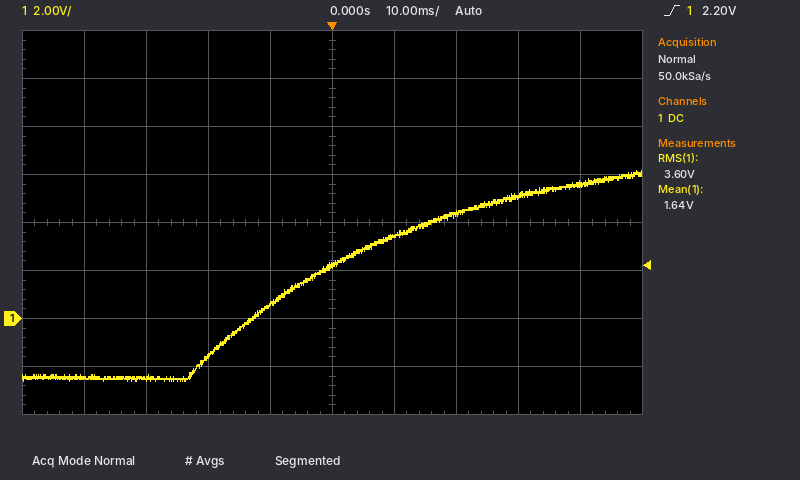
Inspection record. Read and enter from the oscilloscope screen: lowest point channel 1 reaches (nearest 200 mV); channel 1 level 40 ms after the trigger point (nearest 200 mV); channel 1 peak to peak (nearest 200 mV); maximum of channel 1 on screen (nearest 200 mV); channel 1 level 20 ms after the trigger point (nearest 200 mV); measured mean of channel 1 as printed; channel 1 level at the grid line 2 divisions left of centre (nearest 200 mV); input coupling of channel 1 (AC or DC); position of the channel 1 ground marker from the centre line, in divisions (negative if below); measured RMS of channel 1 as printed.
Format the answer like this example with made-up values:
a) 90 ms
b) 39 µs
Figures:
a) -2.6 V
b) 5.6 V
c) 8.8 V
d) 6.2 V
e) 4.4 V
f) 1.64 V
g) -1.6 V
h) DC
i) -2.0 div
j) 3.60 V
